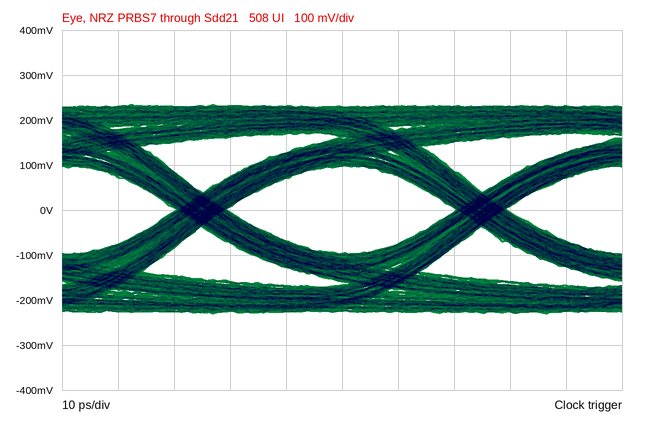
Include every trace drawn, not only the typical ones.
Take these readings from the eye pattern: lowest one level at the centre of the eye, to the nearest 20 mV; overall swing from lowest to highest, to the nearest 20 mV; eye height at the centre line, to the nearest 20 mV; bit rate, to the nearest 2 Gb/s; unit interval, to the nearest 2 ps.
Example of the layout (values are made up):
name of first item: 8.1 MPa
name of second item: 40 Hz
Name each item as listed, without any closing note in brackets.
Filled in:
lowest one level at the centre of the eye, to the nearest 20 mV: 100 mV
overall swing from lowest to highest, to the nearest 20 mV: 460 mV
eye height at the centre line, to the nearest 20 mV: 200 mV
bit rate, to the nearest 2 Gb/s: 20 Gb/s
unit interval, to the nearest 2 ps: 50 ps
